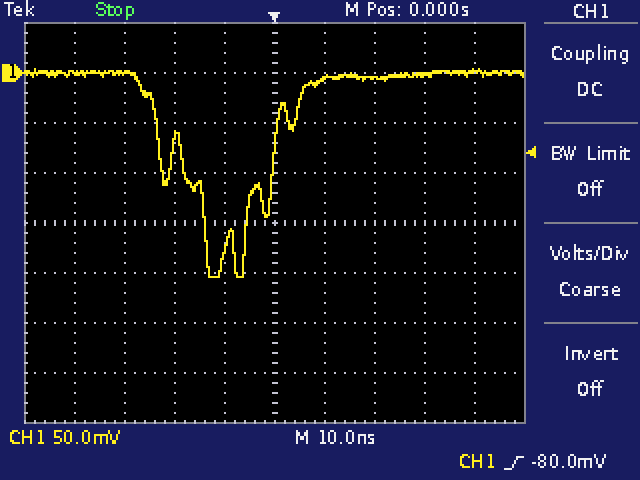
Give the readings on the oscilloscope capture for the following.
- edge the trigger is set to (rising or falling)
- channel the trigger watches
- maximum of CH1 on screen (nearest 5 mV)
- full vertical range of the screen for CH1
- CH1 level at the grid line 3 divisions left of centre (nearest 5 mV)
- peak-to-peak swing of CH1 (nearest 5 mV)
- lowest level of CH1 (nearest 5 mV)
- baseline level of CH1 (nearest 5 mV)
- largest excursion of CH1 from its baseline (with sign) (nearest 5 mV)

rising
CH1
5 mV
400 mV
0 mV
210 mV
-205 mV
0 mV
-205 mV
